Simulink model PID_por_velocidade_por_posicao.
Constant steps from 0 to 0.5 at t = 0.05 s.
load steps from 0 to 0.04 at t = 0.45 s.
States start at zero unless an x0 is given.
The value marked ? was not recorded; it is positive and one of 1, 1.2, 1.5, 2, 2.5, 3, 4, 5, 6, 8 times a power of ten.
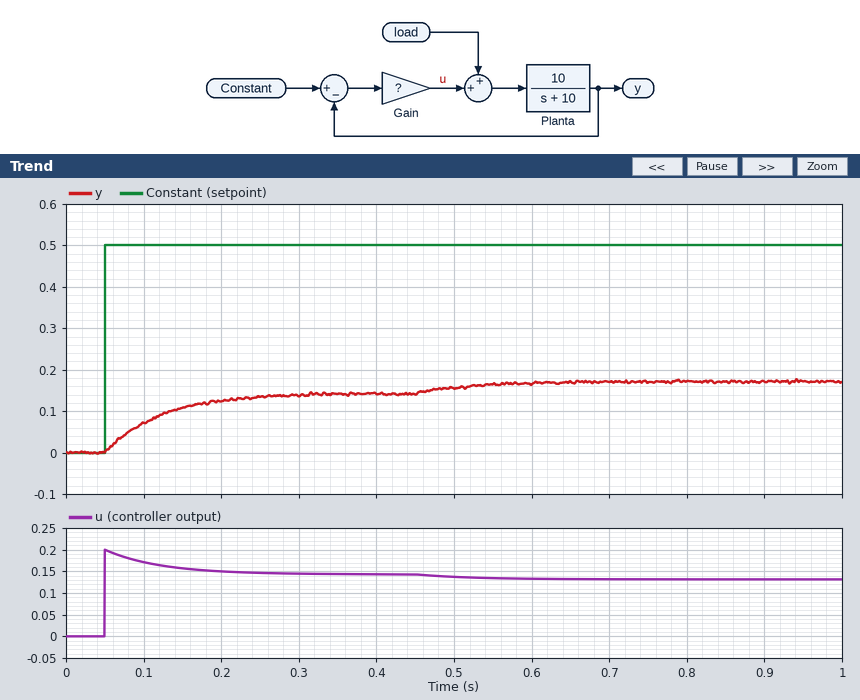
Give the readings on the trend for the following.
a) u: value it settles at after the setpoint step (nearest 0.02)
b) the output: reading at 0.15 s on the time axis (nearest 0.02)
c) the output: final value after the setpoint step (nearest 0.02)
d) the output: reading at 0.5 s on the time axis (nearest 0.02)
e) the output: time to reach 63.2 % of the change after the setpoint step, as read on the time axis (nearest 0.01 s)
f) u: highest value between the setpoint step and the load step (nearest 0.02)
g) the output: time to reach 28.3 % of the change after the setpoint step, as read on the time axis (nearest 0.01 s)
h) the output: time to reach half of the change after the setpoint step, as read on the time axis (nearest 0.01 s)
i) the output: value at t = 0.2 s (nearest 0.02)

0.14
0.10
0.14
0.16
0.12 s
0.20
0.07 s
0.10 s
0.12
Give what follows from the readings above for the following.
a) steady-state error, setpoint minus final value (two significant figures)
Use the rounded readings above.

0.36
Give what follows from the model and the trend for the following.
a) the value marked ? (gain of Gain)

0.4
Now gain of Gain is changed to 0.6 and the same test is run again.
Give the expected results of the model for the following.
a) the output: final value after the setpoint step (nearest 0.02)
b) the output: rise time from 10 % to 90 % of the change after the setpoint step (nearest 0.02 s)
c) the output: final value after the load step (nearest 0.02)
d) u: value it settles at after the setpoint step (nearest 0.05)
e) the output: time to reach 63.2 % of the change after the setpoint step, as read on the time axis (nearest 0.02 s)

0.18
0.14 s
0.22
0.20
0.12 s
